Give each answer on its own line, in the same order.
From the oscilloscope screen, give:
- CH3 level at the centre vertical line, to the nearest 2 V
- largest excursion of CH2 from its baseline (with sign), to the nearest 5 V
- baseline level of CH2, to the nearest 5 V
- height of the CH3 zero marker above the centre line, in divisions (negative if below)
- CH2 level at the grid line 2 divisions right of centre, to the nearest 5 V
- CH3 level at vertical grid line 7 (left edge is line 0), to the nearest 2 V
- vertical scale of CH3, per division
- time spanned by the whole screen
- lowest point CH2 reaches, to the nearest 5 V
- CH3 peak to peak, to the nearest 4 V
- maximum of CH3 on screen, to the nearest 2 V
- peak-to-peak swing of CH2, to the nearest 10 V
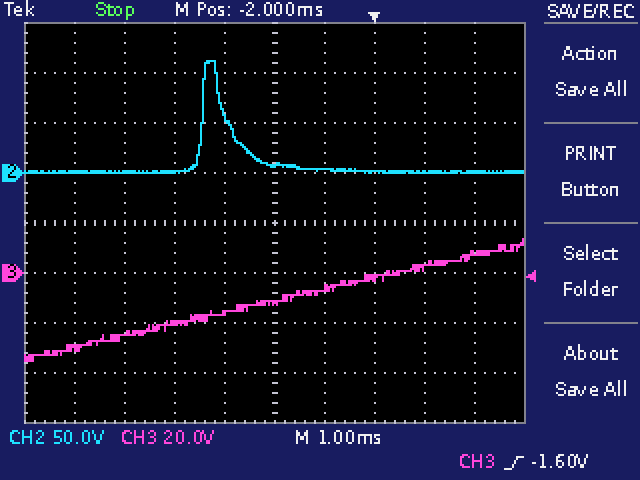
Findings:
-12 V
+110 V
0 V
-1.0 div
0 V
-2 V
20 V
10 ms
0 V
48 V
14 V
110 V
